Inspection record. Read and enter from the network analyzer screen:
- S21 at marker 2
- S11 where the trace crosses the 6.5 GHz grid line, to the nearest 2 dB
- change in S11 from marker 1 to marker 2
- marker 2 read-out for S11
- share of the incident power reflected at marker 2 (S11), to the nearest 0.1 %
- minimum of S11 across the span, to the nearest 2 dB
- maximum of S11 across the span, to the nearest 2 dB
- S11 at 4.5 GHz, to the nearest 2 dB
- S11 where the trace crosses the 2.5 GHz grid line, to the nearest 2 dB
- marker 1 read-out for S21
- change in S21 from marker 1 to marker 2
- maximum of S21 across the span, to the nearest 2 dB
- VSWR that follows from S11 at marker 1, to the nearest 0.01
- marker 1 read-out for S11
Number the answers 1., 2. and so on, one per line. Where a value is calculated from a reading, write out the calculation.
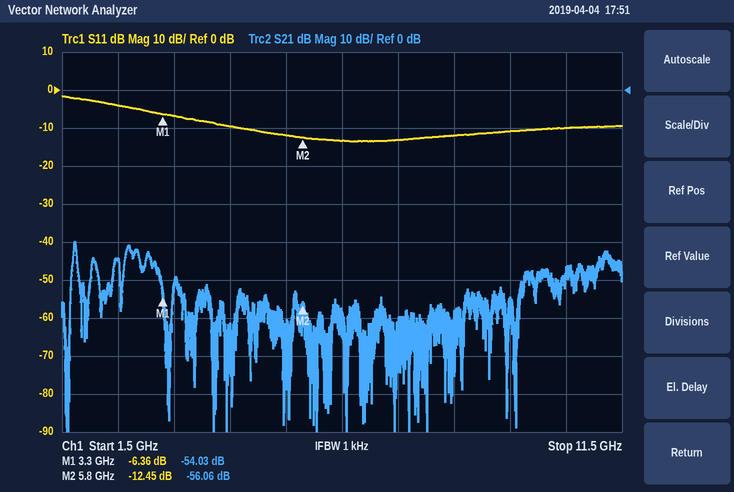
1. -56.06 dB
2. -14 dB
3. -12.45 − (-6.36) = -6.09 dB
4. -12.45 dB
5. 10^(-12.45/10) ≈ 5.7 %
6. -14 dB
7. -2 dB
8. -10 dB
9. -4 dB
10. -54.03 dB
11. -56.06 − (-54.03) = -2.03 dB
12. -40 dB
13. (1 + 0.4808)/(1 − 0.4808) ≈ 2.85
14. -6.36 dB
